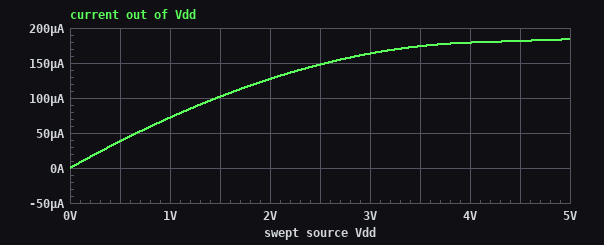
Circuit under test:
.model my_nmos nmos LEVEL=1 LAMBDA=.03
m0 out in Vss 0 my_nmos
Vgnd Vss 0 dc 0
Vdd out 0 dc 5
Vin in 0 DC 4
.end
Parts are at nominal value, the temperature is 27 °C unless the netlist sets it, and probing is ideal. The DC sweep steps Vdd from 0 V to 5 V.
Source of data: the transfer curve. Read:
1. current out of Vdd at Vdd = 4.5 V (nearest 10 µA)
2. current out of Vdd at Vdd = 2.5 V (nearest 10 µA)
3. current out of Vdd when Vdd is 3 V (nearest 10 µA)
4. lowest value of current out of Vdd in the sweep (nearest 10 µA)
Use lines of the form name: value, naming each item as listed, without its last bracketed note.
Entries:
current out of Vdd at Vdd = 4.5 V: 180 µA
current out of Vdd at Vdd = 2.5 V: 150 µA
current out of Vdd when Vdd is 3 V: 160 µA
lowest value of current out of Vdd in the sweep: 0 A
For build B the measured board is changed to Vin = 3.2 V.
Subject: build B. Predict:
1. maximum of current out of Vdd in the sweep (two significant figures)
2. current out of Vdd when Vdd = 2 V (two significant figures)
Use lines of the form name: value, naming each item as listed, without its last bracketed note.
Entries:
maximum of current out of Vdd in the sweep: 120 µA
current out of Vdd when Vdd = 2 V: 93 µA
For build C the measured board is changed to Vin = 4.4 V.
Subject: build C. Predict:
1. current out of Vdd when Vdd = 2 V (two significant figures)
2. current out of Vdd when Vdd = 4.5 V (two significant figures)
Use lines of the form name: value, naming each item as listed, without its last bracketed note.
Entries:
current out of Vdd when Vdd = 2 V: 140 µA
current out of Vdd when Vdd = 4.5 V: 220 µA
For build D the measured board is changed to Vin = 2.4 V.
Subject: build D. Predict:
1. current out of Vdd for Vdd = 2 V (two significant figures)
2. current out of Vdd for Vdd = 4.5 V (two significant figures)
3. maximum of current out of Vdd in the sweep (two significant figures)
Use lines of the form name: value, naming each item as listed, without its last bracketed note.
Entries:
current out of Vdd for Vdd = 2 V: 59 µA
current out of Vdd for Vdd = 4.5 V: 65 µA
maximum of current out of Vdd in the sweep: 66 µA
